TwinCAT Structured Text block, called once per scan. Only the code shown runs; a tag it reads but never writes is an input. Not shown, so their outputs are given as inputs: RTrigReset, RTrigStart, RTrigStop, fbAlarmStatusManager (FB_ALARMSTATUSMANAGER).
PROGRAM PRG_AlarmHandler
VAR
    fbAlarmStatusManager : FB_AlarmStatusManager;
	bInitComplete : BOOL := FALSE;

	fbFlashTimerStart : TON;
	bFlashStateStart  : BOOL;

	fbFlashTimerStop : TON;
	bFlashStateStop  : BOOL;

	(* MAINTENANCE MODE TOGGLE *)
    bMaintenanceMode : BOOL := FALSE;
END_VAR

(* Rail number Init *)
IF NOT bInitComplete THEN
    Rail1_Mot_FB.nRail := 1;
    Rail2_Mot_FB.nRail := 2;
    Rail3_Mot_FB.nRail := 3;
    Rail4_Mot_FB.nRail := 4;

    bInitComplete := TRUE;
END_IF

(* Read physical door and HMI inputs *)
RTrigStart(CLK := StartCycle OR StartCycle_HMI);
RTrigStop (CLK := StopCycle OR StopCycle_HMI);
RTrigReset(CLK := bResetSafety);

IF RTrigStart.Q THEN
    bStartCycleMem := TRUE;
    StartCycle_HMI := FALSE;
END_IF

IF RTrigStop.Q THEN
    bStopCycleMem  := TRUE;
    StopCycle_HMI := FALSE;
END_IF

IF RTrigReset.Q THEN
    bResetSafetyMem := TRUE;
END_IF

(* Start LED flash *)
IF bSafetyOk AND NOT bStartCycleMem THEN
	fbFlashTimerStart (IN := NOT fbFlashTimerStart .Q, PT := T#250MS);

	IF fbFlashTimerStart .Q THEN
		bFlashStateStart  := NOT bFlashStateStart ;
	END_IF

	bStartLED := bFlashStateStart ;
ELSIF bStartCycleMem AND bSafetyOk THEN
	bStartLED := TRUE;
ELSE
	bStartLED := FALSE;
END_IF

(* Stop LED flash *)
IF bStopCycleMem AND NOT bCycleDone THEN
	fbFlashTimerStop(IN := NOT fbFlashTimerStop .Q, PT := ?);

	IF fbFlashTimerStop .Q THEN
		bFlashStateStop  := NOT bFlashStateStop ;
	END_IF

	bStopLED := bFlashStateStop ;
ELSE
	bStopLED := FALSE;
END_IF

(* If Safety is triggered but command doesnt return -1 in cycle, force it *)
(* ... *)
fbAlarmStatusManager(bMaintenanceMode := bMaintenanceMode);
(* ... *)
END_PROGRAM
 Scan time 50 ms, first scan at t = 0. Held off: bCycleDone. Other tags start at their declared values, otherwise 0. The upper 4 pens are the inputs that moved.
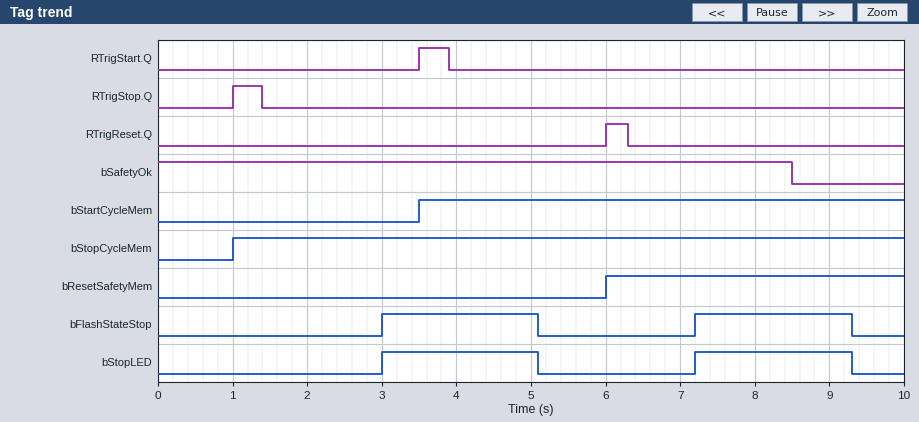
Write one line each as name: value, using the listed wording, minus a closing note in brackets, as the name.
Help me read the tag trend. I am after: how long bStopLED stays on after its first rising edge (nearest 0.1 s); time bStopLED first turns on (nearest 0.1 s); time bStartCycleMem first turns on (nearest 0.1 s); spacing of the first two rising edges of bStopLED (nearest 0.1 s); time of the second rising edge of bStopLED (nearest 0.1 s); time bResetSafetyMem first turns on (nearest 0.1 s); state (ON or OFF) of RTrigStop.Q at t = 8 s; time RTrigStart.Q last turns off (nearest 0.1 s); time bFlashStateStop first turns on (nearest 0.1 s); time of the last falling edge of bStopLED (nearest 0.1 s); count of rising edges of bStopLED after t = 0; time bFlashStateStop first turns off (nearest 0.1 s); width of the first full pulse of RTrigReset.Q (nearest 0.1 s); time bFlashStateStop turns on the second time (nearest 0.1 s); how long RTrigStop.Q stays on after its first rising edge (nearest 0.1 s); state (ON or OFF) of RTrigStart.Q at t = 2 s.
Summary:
how long bStopLED stays on after its first rising edge: 2.1 s
time bStopLED first turns on: 3.0 s
time bStartCycleMem first turns on: 3.5 s
spacing of the first two rising edges of bStopLED: 4.2 s
time of the second rising edge of bStopLED: 7.2 s
time bResetSafetyMem first turns on: 6.0 s
state (ON or OFF) of RTrigStop.Q at t = 8 s: OFF
time RTrigStart.Q last turns off: 3.9 s
time bFlashStateStop first turns on: 3.0 s
time of the last falling edge of bStopLED: 9.3 s
count of rising edges of bStopLED after t = 0: 2
time bFlashStateStop first turns off: 5.1 s
width of the first full pulse of RTrigReset.Q: 0.3 s
time bFlashStateStop turns on the second time: 7.2 s
how long RTrigStop.Q stays on after its first rising edge: 0.4 s
state (ON or OFF) of RTrigStart.Q at t = 2 s: OFF
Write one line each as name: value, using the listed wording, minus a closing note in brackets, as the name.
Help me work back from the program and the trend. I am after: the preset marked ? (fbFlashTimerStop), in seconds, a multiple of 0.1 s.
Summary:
the preset marked ? (fbFlashTimerStop), in seconds, a multiple of 0.1 s: 2.0 s
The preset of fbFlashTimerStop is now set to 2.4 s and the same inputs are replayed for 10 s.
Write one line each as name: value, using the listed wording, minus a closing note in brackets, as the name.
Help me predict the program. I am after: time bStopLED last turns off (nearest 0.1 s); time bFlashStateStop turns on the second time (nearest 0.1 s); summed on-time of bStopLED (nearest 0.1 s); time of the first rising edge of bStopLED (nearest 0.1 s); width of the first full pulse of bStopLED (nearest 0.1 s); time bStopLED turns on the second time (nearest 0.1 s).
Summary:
time bStopLED last turns off: 5.9 s
time bFlashStateStop turns on the second time: 8.4 s
summed on-time of bStopLED: 4.1 s
time of the first rising edge of bStopLED: 3.4 s
width of the first full pulse of bStopLED: 2.5 s
time bStopLED turns on the second time: 8.4 s
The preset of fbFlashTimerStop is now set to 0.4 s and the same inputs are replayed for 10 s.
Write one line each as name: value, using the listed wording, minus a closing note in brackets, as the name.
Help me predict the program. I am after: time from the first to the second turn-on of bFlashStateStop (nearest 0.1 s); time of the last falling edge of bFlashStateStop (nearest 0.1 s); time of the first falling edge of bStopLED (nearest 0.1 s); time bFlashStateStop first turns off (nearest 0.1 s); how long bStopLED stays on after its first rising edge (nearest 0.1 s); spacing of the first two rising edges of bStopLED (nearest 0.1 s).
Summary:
time from the first to the second turn-on of bFlashStateStop: 1.0 s
time of the last falling edge of bFlashStateStop: 9.9 s
time of the first falling edge of bStopLED: 1.9 s
time bFlashStateStop first turns off: 1.9 s
how long bStopLED stays on after its first rising edge: 0.5 s
spacing of the first two rising edges of bStopLED: 1.0 s
